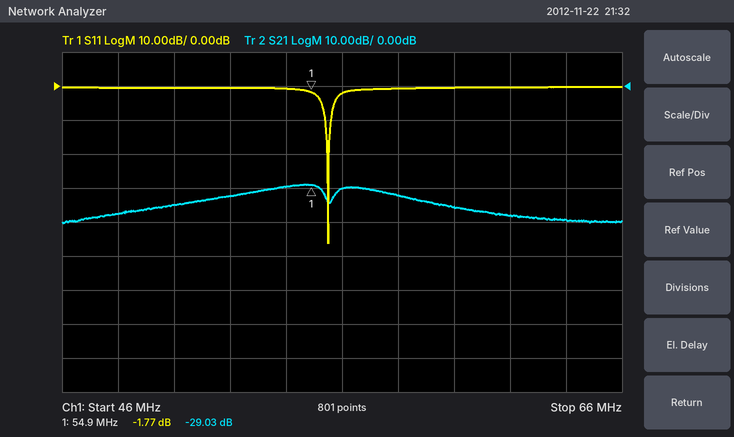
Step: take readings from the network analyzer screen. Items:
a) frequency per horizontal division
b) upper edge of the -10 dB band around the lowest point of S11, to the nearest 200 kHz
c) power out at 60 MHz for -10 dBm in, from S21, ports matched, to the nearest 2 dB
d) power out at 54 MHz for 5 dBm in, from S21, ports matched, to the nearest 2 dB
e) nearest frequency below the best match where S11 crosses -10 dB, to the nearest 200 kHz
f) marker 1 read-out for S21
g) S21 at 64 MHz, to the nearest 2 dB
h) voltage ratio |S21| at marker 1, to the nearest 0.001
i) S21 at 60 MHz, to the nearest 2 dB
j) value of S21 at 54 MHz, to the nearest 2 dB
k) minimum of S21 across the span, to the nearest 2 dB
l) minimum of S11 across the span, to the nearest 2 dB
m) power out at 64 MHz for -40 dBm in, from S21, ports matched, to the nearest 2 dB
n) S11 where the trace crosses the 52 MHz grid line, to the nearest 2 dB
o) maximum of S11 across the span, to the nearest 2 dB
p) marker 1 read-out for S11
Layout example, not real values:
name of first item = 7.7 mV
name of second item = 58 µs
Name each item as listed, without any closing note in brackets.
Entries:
frequency per horizontal division = 2 MHz
upper edge of the -10 dB band around the lowest point of S11, to the nearest 200 kHz = 55.6 MHz
power out at 60 MHz for -10 dBm in, from S21, ports matched, to the nearest 2 dB = -46 dBm
power out at 54 MHz for 5 dBm in, from S21, ports matched, to the nearest 2 dB = -24 dBm
nearest frequency below the best match where S11 crosses -10 dB, to the nearest 200 kHz = 55.4 MHz
marker 1 read-out for S21 = -29.03 dB
S21 at 64 MHz, to the nearest 2 dB = -40 dB
voltage ratio |S21| at marker 1, to the nearest 0.001 = 0.035
S21 at 60 MHz, to the nearest 2 dB = -36 dB
value of S21 at 54 MHz, to the nearest 2 dB = -30 dB
minimum of S21 across the span, to the nearest 2 dB = -40 dB
minimum of S11 across the span, to the nearest 2 dB = -46 dB
power out at 64 MHz for -40 dBm in, from S21, ports matched, to the nearest 2 dB = -80 dBm
S11 where the trace crosses the 52 MHz grid line, to the nearest 2 dB = 0 dB
maximum of S11 across the span, to the nearest 2 dB = 0 dB
marker 1 read-out for S11 = -1.77 dB
